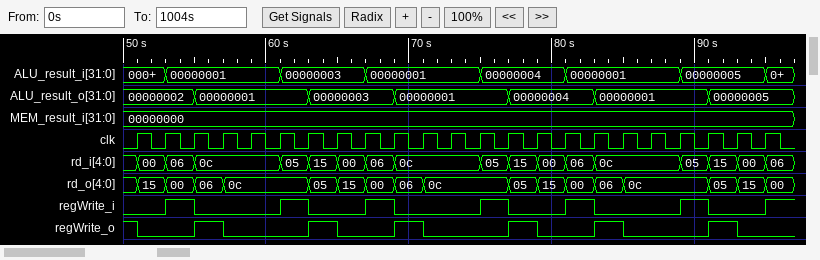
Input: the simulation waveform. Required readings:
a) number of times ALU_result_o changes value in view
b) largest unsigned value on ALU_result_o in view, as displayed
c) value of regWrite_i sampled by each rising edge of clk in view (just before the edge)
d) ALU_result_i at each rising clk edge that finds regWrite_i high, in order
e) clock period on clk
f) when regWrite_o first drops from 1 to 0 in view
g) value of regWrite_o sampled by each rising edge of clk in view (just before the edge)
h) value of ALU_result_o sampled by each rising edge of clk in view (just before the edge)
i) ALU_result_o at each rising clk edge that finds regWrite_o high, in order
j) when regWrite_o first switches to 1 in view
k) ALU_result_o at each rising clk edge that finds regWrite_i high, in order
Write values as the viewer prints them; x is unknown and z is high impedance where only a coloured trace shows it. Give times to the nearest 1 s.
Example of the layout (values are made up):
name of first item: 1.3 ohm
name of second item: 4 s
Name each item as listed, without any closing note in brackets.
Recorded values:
number of times ALU_result_o changes value in view: 6
largest unsigned value on ALU_result_o in view, as displayed: 00000005
value of regWrite_i sampled by each rising edge of clk in view: 0 0 1 0 0 0 1 0 0 1 0 0 0 1 0 0 1 0 0 0 1 0 0
ALU_result_i at each rising clk edge that finds regWrite_i high, in order: 00000001, 00000003, 00000001, 00000004, 00000001, 00000005
clock period on clk: 2 s
when regWrite_o first drops from 1 to 0 in view: 51 s
value of regWrite_o sampled by each rising edge of clk in view: 1 0 0 1 0 0 0 1 0 0 1 0 0 0 1 0 0 1 0 0 0 1 0
value of ALU_result_o sampled by each rising edge of clk in view: 00000002, 00000002, 00000002, 00000001, 00000001, 00000001, 00000001, 00000003, 00000003, 00000003, 00000001, 00000001, 00000001, 00000001, 00000004, 00000004, 00000004, 00000001, 00000001, 00000001, 00000001, 00000005, 00000005
ALU_result_o at each rising clk edge that finds regWrite_o high, in order: 00000002, 00000001, 00000003, 00000001, 00000004, 00000001, 00000005
when regWrite_o first switches to 1 in view: 55 s
ALU_result_o at each rising clk edge that finds regWrite_i high, in order: 00000002, 00000001, 00000003, 00000001, 00000004, 00000001
